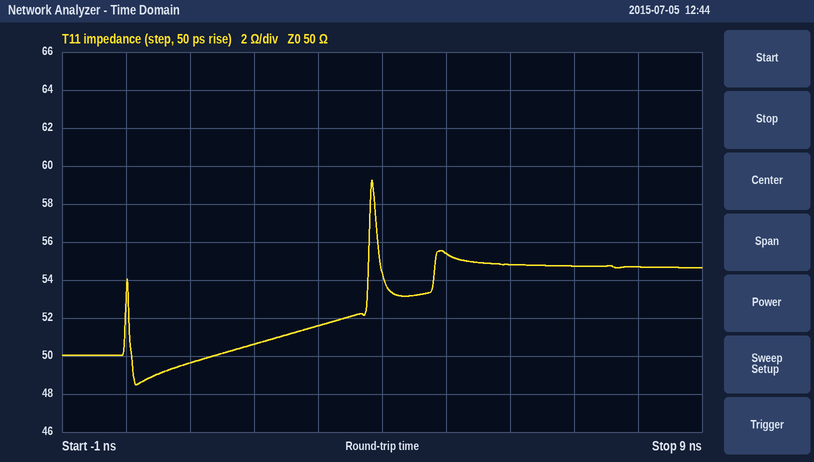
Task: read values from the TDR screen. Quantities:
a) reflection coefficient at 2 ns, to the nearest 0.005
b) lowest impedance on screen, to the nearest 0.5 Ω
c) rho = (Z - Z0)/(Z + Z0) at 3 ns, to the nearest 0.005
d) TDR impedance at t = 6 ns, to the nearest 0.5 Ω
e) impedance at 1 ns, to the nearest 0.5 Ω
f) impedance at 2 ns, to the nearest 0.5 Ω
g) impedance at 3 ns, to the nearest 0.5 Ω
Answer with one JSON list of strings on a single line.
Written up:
["+0.005", "48.5 Ω", "+0.015", "55.0 Ω", "49.5 Ω", "50.5 Ω", "51.5 Ω"]
